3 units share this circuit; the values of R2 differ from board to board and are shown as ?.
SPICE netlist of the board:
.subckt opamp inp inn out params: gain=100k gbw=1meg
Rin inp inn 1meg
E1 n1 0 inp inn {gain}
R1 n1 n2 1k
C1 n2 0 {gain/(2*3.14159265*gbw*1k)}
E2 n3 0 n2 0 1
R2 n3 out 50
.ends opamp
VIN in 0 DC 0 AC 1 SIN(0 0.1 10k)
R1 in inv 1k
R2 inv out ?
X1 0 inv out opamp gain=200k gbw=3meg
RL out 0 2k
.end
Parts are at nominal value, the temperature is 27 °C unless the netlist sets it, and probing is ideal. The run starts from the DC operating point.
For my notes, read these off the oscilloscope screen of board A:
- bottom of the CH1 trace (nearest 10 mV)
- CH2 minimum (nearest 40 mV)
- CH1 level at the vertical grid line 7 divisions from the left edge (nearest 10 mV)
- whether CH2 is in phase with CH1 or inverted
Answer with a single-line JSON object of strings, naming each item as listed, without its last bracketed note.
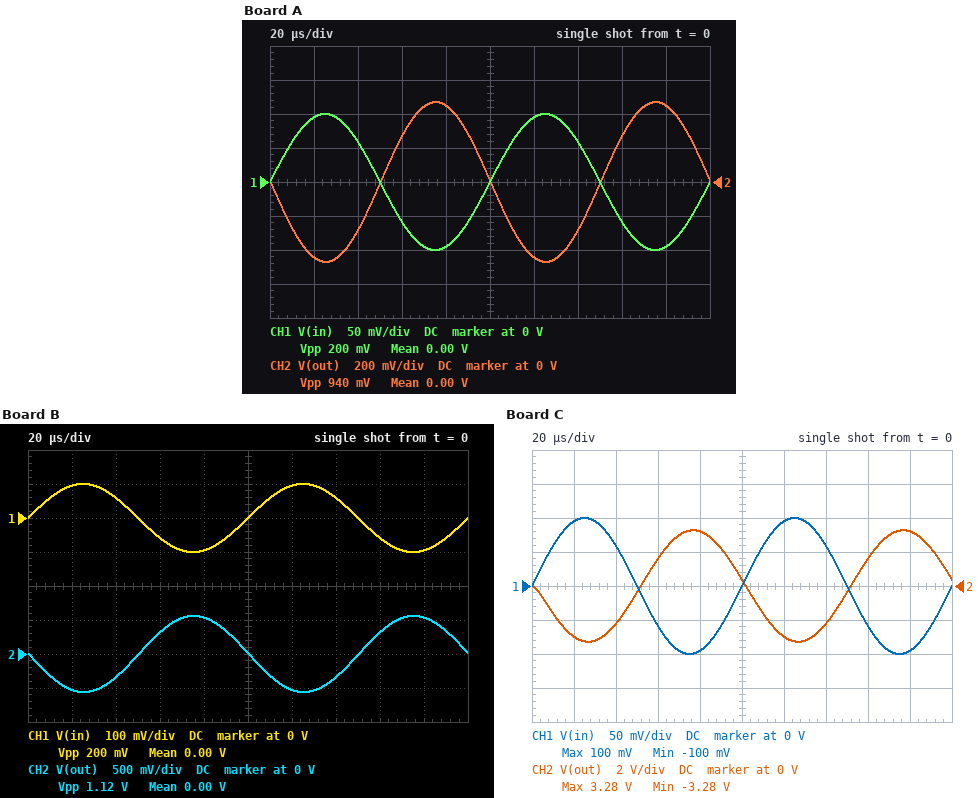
{"bottom of the CH1 trace": "-100 mV", "CH2 minimum": "-480 mV", "CH1 level at the vertical grid line 7 divisions from the left edge": "60 mV", "whether CH2 is in phase with CH1 or inverted": "inverted"}
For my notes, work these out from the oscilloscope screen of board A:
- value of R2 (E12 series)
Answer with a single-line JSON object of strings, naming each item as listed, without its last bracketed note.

{"value of R2": "4.7 kΩ"}
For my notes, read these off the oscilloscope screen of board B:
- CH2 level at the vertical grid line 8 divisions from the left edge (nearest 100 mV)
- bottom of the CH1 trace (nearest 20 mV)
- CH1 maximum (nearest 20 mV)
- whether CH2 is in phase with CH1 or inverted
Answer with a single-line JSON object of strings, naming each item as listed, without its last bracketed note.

{"CH2 level at the vertical grid line 8 divisions from the left edge": "300 mV", "bottom of the CH1 trace": "-100 mV", "CH1 maximum": "100 mV", "whether CH2 is in phase with CH1 or inverted": "inverted"}
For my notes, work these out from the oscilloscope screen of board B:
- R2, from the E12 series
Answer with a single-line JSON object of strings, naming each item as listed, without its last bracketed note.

{"R2, from the E12 series": "5.6 kΩ"}
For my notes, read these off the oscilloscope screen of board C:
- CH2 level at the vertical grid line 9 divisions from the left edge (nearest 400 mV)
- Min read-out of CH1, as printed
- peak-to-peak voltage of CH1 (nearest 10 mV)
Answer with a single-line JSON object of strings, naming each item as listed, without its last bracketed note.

{"CH2 level at the vertical grid line 9 divisions from the left edge": "3.2 V", "Min read-out of CH1, as printed": "-100 mV", "peak-to-peak voltage of CH1": "200 mV"}
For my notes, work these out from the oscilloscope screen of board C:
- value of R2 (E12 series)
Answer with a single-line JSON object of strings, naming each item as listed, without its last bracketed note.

{"value of R2": "33 kΩ"}
